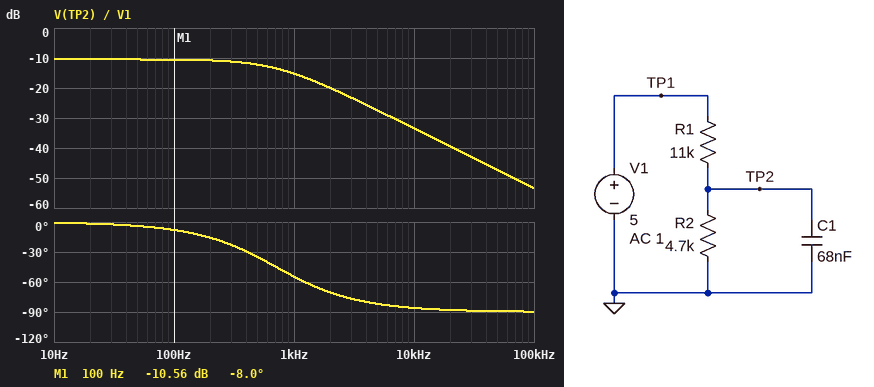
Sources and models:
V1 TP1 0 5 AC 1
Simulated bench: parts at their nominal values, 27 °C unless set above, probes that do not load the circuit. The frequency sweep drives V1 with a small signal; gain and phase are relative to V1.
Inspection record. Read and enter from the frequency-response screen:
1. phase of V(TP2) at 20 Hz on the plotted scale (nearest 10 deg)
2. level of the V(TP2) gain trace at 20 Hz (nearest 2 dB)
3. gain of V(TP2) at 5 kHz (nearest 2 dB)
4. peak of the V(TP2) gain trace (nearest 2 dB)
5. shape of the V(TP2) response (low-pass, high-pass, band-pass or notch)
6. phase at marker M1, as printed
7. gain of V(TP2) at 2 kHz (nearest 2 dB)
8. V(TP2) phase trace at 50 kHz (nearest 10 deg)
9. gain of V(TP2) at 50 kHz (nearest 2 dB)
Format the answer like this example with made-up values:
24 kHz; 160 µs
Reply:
0 deg; -10 dB; -28 dB; -10 dB; low-pass; -8.0 deg; -20 dB; -90 deg; -48 dB
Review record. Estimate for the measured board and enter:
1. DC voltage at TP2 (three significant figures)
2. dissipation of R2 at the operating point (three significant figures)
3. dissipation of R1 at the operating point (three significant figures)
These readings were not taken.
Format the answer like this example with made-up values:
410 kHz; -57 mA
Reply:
1.50 V; 477 µW; 1.12 mW
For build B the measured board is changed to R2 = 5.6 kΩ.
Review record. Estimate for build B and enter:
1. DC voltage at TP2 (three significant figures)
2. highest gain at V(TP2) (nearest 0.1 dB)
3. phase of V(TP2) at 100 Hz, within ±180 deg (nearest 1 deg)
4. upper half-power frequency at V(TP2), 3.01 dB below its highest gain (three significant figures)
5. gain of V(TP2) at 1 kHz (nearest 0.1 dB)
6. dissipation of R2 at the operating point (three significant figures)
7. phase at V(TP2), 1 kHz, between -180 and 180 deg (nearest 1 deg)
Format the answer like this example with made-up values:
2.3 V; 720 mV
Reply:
1.69 V; -9.4 dB; -9 deg; 631 Hz; -14.9 dB; 508 µW; -58 deg
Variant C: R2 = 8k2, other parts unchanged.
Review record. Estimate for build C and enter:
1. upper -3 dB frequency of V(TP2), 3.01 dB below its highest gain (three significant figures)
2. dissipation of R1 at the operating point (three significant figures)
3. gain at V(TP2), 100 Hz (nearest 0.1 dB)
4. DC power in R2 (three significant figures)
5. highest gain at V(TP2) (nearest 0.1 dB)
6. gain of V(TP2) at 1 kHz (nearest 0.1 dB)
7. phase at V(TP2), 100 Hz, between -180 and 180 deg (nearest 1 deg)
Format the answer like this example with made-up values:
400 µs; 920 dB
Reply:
498 Hz; 746 µW; -7.6 dB; 556 µW; -7.4 dB; -14.4 dB; -11 deg
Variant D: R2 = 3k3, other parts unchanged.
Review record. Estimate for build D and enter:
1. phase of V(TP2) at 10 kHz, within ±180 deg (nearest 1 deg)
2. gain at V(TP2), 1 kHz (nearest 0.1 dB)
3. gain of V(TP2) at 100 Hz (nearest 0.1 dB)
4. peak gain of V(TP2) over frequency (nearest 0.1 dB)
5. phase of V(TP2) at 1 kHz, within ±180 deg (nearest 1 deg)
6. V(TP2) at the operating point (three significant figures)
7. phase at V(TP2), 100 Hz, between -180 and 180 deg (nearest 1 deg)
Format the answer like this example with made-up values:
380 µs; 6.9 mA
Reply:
-85 deg; -16.1 dB; -12.8 dB; -12.7 dB; -47 deg; 1.15 V; -6 deg
